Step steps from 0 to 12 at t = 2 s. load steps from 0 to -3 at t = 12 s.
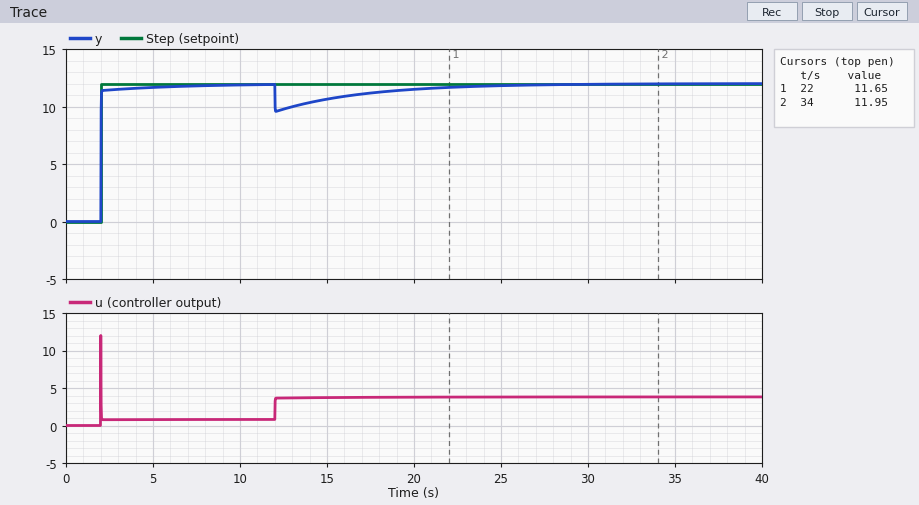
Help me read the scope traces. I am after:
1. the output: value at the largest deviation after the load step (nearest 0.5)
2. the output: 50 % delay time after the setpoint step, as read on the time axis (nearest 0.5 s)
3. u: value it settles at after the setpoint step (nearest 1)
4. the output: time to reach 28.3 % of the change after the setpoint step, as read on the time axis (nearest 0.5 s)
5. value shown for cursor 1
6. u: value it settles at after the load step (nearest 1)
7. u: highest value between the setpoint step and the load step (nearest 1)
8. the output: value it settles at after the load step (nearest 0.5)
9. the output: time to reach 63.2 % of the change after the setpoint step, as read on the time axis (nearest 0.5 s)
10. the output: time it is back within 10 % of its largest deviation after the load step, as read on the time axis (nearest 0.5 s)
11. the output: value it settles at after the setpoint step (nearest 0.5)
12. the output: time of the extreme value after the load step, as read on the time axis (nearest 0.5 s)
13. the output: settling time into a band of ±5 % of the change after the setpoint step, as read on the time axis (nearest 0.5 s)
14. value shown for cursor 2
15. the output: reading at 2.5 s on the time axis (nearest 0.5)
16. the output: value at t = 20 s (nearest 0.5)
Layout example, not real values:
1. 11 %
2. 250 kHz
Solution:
1. 9.5
2. 2.0 s
3. 1
4. 2.0 s
5. 11.65
6. 4
7. 12
8. 12.0
9. 2.0 s
10. 24.0 s
11. 12.0
12. 12.0 s
13. 2.0 s
14. 11.95
15. 11.5
16. 11.5
